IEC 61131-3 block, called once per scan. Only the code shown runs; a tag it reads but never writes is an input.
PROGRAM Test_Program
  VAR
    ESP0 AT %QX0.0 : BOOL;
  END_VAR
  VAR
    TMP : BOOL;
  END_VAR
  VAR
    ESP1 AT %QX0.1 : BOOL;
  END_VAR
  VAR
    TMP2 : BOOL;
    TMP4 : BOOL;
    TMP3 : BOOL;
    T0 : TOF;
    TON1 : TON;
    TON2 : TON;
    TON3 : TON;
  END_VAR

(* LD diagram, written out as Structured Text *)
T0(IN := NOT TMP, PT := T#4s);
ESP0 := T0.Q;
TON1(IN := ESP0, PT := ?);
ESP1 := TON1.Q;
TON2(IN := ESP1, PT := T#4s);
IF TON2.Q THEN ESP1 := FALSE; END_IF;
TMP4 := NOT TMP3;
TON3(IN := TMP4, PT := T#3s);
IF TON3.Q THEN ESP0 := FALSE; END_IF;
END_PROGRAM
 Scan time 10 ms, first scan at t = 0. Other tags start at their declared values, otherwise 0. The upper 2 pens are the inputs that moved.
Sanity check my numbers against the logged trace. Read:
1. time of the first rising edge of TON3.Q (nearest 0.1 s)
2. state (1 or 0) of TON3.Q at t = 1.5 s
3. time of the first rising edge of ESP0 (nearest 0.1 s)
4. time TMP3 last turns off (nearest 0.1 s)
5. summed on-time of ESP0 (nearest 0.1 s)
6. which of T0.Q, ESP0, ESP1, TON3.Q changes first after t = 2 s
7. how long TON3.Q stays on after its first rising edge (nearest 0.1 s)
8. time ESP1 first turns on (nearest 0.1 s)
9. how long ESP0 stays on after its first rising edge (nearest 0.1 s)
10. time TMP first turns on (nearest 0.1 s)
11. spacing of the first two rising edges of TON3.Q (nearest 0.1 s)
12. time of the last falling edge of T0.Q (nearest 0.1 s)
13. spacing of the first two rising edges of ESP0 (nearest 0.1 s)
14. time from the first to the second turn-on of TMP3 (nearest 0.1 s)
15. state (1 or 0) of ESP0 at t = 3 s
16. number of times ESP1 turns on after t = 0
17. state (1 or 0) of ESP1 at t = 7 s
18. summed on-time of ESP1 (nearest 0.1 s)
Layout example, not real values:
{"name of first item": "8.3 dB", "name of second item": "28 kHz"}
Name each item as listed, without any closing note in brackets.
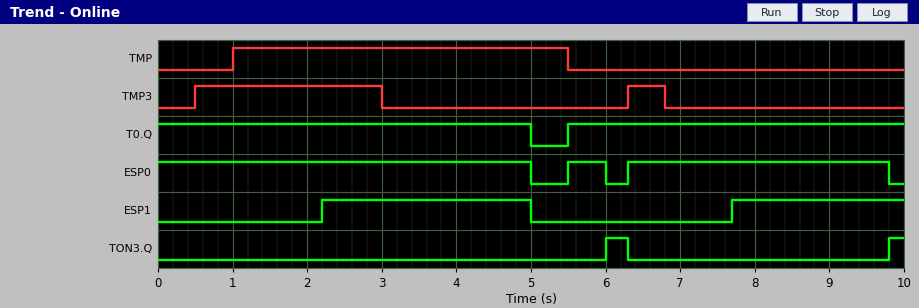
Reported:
{"time of the first rising edge of TON3.Q": "6.0 s", "state (1 or 0) of TON3.Q at t = 1.5 s": "0", "time of the first rising edge of ESP0": "5.5 s", "time TMP3 last turns off": "6.8 s", "summed on-time of ESP0": "9.0 s", "which of T0.Q, ESP0, ESP1, TON3.Q changes first after t = 2 s": "ESP1", "how long TON3.Q stays on after its first rising edge": "0.3 s", "time ESP1 first turns on": "2.2 s", "how long ESP0 stays on after its first rising edge": "0.5 s", "time TMP first turns on": "1.0 s", "spacing of the first two rising edges of TON3.Q": "3.8 s", "time of the last falling edge of T0.Q": "5.0 s", "spacing of the first two rising edges of ESP0": "0.8 s", "time from the first to the second turn-on of TMP3": "5.8 s", "state (1 or 0) of ESP0 at t = 3 s": "1", "number of times ESP1 turns on after t = 0": "2", "state (1 or 0) of ESP1 at t = 7 s": "0", "summed on-time of ESP1": "5.1 s"}
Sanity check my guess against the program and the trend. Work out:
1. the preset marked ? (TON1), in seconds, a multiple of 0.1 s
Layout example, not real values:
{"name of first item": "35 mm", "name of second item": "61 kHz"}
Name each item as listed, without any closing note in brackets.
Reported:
{"the preset marked ? (TON1), in seconds, a multiple of 0.1 s": "2.2 s"}
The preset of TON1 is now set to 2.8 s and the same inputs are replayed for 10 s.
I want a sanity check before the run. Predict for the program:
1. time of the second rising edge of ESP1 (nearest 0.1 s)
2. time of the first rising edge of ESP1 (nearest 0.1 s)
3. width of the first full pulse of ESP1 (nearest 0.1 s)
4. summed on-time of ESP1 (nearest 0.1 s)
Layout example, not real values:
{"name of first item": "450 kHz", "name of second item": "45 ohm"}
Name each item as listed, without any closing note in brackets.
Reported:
{"time of the second rising edge of ESP1": "8.3 s", "time of the first rising edge of ESP1": "2.8 s", "width of the first full pulse of ESP1": "2.2 s", "summed on-time of ESP1": "3.9 s"}
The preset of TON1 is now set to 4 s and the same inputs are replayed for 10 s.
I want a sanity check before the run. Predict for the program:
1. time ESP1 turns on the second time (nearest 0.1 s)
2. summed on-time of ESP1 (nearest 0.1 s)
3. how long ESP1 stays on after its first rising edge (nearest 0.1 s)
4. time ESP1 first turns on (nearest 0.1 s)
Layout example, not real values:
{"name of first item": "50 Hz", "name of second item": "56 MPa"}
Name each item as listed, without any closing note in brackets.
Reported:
{"time ESP1 turns on the second time": "9.5 s", "summed on-time of ESP1": "1.5 s", "how long ESP1 stays on after its first rising edge": "1.0 s", "time ESP1 first turns on": "4.0 s"}
